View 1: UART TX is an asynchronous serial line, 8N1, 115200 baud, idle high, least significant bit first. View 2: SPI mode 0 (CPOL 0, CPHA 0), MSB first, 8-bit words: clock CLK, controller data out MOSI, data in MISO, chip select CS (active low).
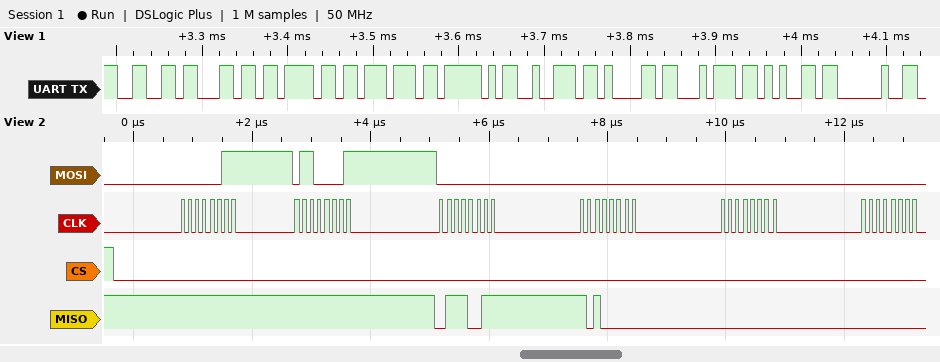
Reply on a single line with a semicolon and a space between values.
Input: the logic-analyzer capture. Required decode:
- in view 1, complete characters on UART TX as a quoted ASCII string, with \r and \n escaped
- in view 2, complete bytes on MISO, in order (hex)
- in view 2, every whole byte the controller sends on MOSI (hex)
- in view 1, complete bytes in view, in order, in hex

"flow_rate "; FF FF 73 A0 00 00; 03 61 00 00 00 00; 66 6C 6F 77 5F 72 61 74 65 20
